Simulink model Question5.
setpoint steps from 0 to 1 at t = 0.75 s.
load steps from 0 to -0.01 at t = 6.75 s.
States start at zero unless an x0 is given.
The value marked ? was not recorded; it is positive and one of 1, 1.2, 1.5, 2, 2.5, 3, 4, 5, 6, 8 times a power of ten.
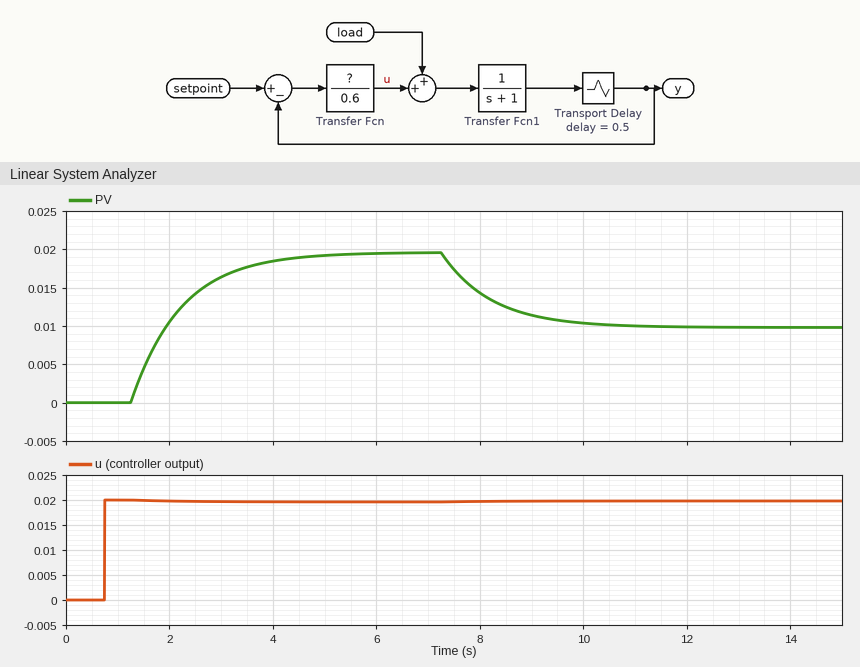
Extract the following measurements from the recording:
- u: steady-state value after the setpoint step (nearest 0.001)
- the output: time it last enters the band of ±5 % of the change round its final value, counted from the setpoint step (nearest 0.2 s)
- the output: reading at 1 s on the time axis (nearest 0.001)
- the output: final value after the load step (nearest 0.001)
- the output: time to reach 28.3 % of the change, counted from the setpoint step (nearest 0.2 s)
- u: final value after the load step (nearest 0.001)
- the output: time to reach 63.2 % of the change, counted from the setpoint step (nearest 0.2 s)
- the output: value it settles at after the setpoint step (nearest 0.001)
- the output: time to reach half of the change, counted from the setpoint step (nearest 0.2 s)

0.020
3.4 s
0.000
0.010
0.8 s
0.020
1.4 s
0.020
1.2 s
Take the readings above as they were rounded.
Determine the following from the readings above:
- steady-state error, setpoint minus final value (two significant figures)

0.98
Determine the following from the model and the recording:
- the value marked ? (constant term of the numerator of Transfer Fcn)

0.012
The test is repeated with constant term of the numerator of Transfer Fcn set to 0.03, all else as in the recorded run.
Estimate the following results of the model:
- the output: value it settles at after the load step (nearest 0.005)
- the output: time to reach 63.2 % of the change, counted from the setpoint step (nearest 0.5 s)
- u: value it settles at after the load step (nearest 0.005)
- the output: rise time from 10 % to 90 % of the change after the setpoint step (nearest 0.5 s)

0.040
1.5 s
0.050
2.0 s
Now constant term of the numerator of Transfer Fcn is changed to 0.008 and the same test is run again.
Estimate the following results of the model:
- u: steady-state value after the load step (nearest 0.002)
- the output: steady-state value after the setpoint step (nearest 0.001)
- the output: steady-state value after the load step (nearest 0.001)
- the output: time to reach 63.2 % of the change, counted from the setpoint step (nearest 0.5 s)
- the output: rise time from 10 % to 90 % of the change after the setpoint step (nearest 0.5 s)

0.014
0.013
0.003
1.5 s
2.0 s
